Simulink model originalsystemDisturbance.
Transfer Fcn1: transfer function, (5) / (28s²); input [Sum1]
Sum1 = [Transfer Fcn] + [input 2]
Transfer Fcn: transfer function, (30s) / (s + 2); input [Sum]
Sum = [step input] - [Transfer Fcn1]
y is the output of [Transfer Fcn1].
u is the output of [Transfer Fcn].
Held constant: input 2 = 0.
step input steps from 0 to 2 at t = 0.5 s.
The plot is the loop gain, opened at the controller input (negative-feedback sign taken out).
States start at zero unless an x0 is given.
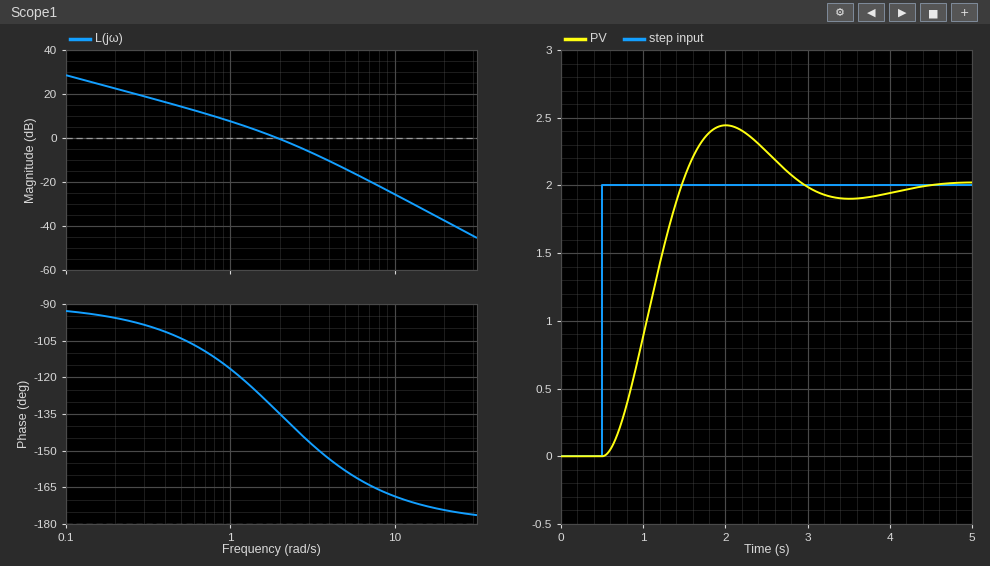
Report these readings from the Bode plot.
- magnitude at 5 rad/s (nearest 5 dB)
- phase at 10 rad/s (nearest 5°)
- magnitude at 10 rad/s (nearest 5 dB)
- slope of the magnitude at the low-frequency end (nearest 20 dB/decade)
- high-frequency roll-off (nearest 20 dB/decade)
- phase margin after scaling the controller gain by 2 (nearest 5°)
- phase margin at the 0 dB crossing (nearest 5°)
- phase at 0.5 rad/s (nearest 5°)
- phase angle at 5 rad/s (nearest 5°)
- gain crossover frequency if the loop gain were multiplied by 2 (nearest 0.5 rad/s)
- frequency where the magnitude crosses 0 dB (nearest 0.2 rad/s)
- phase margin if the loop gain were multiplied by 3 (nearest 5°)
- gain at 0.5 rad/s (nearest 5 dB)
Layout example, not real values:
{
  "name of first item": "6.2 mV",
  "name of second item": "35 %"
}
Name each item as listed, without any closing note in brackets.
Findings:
{
  "magnitude at 5 rad/s": "-15 dB",
  "phase at 10 rad/s": "-170°",
  "magnitude at 10 rad/s": "-25 dB",
  "slope of the magnitude at the low-frequency end": "-20 dB/decade",
  "high-frequency roll-off": "-40 dB/decade",
  "phase margin after scaling the controller gain by 2": "35°",
  "phase margin at the 0 dB crossing": "45°",
  "phase at 0.5 rad/s": "-105°",
  "phase angle at 5 rad/s": "-160°",
  "gain crossover frequency if the loop gain were multiplied by 2": "3.0 rad/s",
  "frequency where the magnitude crosses 0 dB": "2.0 rad/s",
  "phase margin if the loop gain were multiplied by 3": "30°",
  "gain at 0.5 rad/s": "15 dB"
}
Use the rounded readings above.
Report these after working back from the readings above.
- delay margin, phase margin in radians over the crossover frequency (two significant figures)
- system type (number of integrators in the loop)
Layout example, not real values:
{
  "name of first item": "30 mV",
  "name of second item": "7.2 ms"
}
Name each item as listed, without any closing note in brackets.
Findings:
{
  "delay margin, phase margin in radians over the crossover frequency": "0.39 s",
  "system type": "1"
}
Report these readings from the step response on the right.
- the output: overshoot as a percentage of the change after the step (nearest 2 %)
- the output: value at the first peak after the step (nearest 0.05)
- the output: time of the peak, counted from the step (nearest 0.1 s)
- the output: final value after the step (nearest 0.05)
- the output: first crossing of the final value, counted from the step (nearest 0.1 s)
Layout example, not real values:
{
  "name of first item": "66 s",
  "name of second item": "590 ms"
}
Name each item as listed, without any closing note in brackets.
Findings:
{
  "the output: overshoot as a percentage of the change after the step": "22 %",
  "the output: value at the first peak after the step": "2.45",
  "the output: time of the peak, counted from the step": "1.5 s",
  "the output: final value after the step": "2.00",
  "the output: first crossing of the final value, counted from the step": "1.0 s"
}
